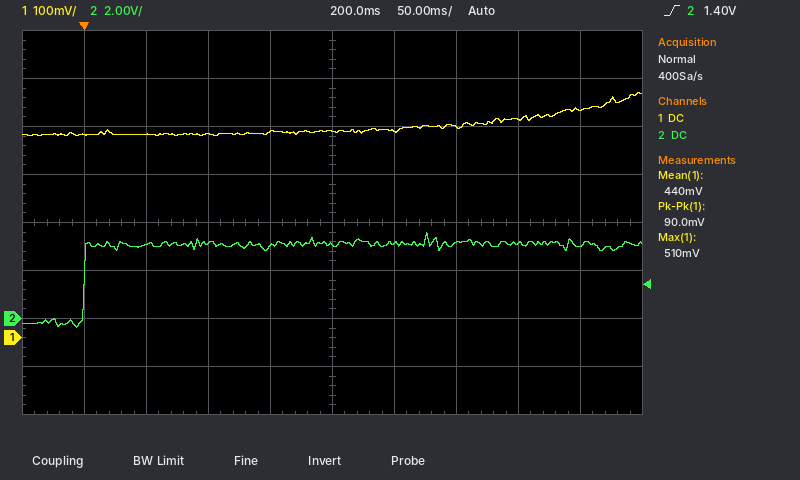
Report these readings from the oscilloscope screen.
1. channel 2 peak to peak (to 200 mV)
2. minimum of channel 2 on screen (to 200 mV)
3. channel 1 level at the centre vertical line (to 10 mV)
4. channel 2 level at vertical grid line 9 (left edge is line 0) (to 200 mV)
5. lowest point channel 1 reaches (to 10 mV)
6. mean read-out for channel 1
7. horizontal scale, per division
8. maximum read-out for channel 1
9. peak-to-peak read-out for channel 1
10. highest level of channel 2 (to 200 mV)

4.0 V
-400 mV
430 mV
3.0 V
420 mV
440 mV
50 ms
510 mV
90.0 mV
3.6 V
